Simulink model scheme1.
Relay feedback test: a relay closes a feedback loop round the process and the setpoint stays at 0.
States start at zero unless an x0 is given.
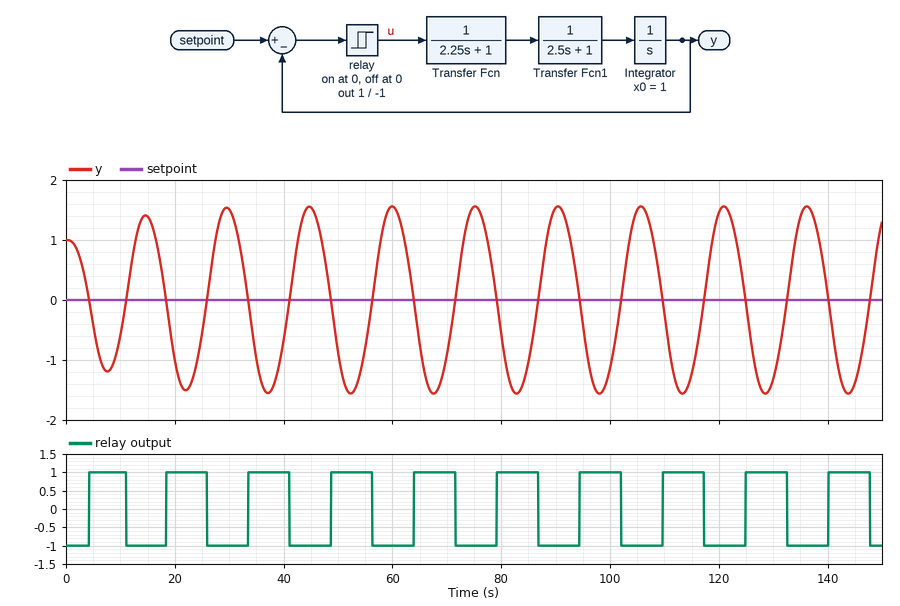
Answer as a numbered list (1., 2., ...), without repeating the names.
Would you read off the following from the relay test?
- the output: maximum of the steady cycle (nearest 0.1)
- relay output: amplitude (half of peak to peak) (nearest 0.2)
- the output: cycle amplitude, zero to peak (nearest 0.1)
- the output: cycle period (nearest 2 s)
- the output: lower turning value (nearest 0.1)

1. 1.6
2. 1.0
3. 1.6
4. 16 s
5. -1.6
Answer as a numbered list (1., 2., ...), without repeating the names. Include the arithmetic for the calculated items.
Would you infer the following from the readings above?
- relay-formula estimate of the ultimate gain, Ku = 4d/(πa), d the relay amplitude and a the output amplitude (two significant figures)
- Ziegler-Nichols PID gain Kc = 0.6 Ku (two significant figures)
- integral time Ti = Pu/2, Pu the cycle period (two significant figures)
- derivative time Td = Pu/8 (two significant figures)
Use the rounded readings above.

1. 4 × 1 / (π × 1.6) = 0.80
2. 0.6 × 0.8 = 0.48
3. 16 / 2 = 8.0 s
4. 16 / 8 = 2.0 s
